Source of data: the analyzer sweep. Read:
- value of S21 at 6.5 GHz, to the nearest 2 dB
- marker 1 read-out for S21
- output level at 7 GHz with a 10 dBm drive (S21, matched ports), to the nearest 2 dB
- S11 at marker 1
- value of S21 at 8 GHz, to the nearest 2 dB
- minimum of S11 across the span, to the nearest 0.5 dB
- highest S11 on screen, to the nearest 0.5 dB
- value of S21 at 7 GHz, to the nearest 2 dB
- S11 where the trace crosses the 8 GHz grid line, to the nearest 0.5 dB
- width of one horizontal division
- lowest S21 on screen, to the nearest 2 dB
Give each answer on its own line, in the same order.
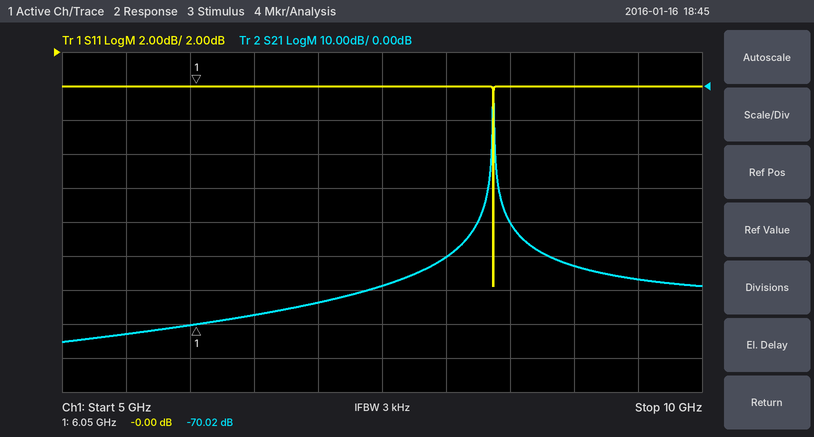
-68 dB
-70.02 dB
-54 dBm
-0.00 dB
-50 dB
-12.0 dB
0.0 dB
-64 dB
0.0 dB
500 MHz
-76 dB
